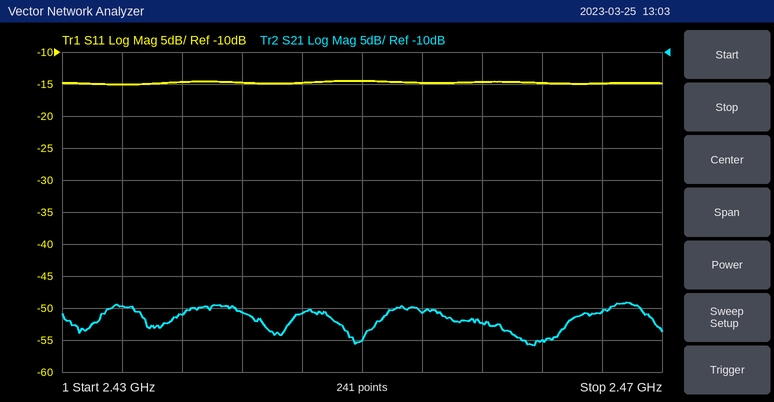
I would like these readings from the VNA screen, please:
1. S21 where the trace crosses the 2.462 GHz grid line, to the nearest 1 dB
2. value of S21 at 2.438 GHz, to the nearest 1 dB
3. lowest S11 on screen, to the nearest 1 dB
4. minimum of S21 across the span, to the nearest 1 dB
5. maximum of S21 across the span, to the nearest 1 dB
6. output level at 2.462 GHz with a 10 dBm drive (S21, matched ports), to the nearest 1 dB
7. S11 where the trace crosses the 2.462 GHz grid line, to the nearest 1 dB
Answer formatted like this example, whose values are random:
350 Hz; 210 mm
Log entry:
-55 dB; -51 dB; -15 dB; -56 dB; -49 dB; -45 dBm; -15 dB
